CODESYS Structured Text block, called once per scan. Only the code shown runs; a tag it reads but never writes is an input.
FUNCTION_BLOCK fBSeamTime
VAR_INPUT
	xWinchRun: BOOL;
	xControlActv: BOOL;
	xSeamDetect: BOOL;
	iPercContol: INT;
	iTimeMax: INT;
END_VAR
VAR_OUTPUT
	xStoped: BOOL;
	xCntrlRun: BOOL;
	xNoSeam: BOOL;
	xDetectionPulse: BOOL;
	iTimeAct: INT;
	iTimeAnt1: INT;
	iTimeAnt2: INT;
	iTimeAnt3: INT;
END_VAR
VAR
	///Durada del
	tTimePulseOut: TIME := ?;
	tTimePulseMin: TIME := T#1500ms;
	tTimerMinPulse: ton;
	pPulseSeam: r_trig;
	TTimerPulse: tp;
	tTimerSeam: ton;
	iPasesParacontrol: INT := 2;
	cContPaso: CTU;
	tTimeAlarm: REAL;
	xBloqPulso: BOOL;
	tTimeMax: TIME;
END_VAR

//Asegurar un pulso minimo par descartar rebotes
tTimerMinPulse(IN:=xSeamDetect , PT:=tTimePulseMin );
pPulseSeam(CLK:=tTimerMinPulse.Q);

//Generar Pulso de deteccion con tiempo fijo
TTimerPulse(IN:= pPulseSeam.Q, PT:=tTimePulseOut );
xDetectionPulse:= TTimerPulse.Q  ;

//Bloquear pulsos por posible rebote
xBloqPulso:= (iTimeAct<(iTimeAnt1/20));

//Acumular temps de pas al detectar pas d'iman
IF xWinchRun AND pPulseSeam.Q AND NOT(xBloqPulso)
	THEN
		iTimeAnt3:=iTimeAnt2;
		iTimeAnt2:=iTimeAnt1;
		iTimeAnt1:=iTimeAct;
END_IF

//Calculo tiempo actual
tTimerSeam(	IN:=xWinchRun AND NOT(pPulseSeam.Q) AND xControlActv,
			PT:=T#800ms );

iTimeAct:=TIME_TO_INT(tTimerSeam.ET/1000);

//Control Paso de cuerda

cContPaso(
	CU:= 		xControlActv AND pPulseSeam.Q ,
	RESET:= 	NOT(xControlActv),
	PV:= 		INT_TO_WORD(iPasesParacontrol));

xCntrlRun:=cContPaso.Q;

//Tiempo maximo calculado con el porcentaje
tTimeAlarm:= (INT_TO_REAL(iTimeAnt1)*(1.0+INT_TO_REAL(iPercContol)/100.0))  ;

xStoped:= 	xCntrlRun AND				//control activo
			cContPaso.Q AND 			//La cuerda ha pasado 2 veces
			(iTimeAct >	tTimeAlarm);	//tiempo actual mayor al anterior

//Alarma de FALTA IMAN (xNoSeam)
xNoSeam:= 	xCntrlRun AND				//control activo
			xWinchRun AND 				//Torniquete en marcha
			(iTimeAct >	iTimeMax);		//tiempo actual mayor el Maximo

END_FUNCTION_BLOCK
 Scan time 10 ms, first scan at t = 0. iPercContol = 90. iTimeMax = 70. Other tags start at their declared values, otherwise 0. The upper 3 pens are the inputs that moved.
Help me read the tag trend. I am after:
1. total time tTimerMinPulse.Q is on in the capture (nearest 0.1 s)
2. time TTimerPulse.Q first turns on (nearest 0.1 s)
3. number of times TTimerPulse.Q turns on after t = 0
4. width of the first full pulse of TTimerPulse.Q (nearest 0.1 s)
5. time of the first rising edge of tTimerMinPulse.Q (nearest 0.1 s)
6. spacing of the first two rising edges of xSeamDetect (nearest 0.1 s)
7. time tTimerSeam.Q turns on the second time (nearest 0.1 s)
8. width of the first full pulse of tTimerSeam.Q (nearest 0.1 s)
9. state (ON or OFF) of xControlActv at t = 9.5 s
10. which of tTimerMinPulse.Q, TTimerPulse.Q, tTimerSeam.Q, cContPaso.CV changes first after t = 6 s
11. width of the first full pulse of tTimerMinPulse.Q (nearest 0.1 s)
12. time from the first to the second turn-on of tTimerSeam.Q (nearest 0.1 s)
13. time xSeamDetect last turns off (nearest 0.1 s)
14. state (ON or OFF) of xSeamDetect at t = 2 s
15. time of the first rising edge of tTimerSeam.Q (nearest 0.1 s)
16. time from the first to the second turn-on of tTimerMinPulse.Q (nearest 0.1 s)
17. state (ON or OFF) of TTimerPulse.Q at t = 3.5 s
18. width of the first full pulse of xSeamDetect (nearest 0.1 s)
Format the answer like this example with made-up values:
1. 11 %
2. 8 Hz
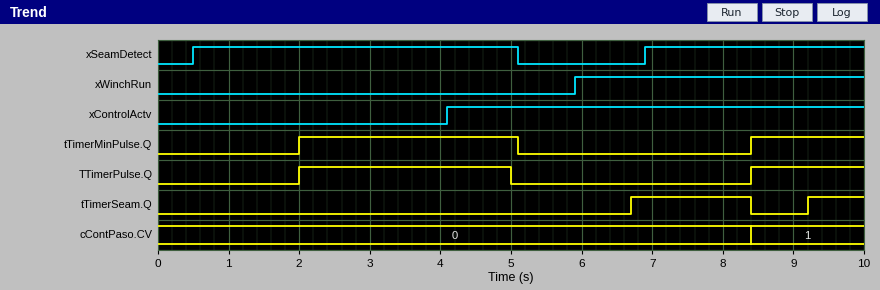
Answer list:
1. 4.7 s
2. 2.0 s
3. 2
4. 3.0 s
5. 2.0 s
6. 6.4 s
7. 9.2 s
8. 1.7 s
9. ON
10. tTimerSeam.Q
11. 3.1 s
12. 2.5 s
13. 5.1 s
14. ON
15. 6.7 s
16. 6.4 s
17. ON
18. 4.6 s
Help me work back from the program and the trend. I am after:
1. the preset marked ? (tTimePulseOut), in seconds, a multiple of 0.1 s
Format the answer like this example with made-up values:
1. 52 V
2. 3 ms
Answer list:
1. 3.0 s
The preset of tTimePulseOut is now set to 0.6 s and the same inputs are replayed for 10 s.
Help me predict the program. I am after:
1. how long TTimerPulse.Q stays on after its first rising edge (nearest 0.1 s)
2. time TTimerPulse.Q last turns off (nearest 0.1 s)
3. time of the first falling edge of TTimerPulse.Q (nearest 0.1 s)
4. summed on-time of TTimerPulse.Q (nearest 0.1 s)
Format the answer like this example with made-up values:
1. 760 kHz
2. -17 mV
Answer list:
1. 0.6 s
2. 9.0 s
3. 2.6 s
4. 1.2 s
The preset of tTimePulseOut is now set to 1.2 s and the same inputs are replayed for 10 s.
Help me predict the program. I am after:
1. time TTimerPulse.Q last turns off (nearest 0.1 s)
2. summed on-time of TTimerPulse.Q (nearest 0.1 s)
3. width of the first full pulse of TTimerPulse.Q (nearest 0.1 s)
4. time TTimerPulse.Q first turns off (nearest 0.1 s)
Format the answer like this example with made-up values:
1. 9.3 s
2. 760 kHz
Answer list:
1. 9.6 s
2. 2.4 s
3. 1.2 s
4. 3.2 s
